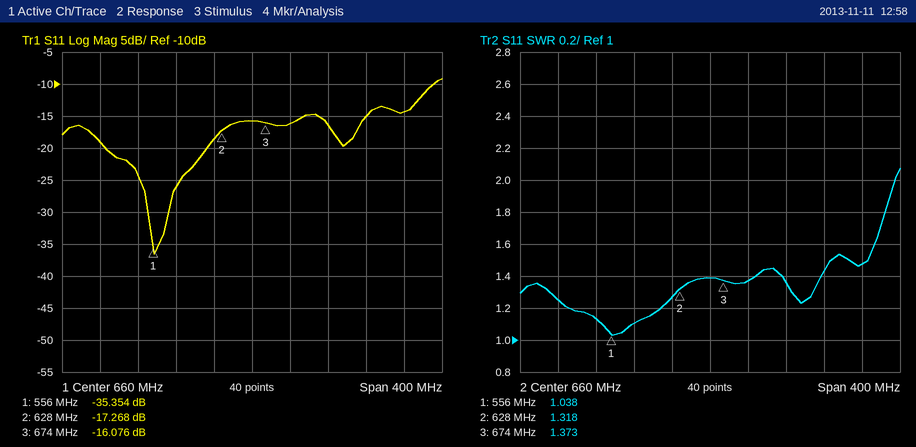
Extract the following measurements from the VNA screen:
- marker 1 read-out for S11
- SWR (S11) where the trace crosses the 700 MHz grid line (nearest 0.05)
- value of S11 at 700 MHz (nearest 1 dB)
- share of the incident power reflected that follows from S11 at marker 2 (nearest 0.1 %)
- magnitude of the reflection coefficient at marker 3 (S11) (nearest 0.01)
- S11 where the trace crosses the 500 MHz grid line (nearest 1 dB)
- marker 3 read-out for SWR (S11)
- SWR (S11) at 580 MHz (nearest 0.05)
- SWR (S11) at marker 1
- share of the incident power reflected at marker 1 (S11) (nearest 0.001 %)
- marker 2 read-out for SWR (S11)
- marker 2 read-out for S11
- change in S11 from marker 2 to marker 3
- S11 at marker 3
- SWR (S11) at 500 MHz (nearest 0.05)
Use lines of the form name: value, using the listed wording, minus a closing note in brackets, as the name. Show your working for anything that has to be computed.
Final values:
marker 1 read-out for S11: -35.354 dB
SWR (S11) where the trace crosses the 700 MHz grid line: 1.35
value of S11 at 700 MHz: -16 dB
share of the incident power reflected that follows from S11 at marker 2: 10^(-17.268/10) ≈ 1.9 %
magnitude of the reflection coefficient at marker 3 (S11): 10^(-16.076/20) ≈ 0.16
S11 where the trace crosses the 500 MHz grid line: -19 dB
marker 3 read-out for SWR: 1.373
SWR (S11) at 580 MHz: 1.10
SWR (S11) at marker 1: 1.038
share of the incident power reflected at marker 1 (S11): 10^(-35.354/10) ≈ 0.029 %
marker 2 read-out for SWR: 1.318
marker 2 read-out for S11: -17.268 dB
change in S11 from marker 2 to marker 3: -16.076 − (-17.268) = 1.192 dB
S11 at marker 3: -16.076 dB
SWR (S11) at 500 MHz: 1.25
